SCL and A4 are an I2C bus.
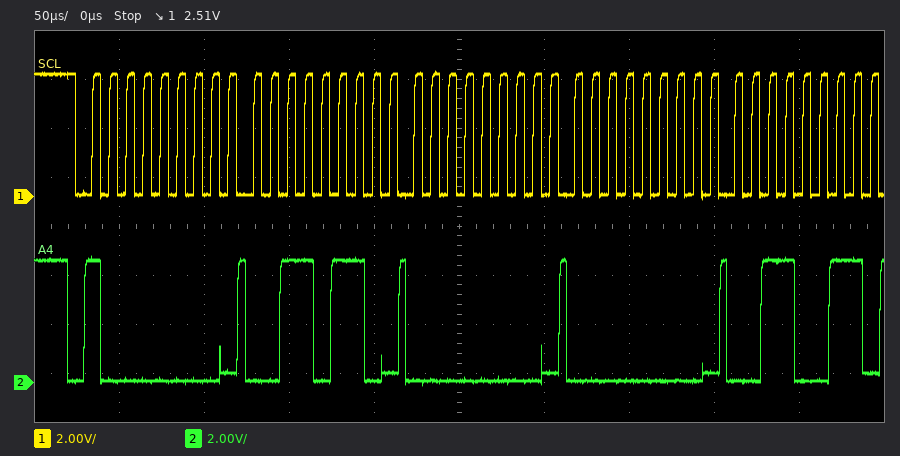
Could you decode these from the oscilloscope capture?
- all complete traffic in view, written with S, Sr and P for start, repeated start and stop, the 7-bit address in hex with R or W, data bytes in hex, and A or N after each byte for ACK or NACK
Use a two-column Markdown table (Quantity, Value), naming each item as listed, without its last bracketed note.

| Quantity | Value |
|---|---|
| all complete traffic in view, written with S, Sr and P for start, repeated start and stop, the 7-bit address in hex with R or W, data bytes in hex, and A or N after each byte for ACK or NACK | S 40W A 36 A 00 A 00 A 33 A |
